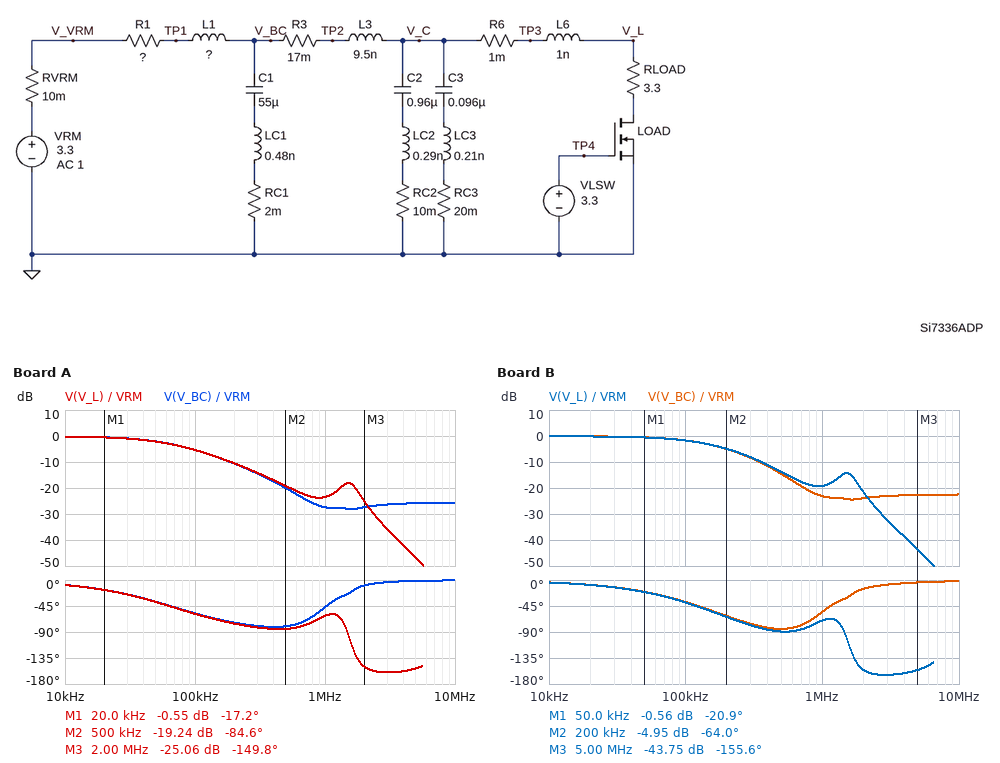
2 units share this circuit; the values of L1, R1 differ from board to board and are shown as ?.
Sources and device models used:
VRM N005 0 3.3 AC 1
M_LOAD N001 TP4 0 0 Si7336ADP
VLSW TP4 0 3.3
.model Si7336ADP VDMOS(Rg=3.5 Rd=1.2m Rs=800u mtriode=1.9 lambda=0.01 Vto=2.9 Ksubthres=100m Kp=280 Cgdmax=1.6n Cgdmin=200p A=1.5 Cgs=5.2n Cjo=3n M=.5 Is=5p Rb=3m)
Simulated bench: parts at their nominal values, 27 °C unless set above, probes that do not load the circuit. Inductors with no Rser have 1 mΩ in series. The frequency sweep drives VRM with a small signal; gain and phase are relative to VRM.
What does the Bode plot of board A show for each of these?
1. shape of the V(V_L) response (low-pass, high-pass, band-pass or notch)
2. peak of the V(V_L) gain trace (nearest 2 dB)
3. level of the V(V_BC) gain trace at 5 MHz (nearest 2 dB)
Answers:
low-pass
0 dB
-26 dB
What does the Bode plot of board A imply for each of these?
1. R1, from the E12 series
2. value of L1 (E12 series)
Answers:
0.033 Ω
8.2 nH
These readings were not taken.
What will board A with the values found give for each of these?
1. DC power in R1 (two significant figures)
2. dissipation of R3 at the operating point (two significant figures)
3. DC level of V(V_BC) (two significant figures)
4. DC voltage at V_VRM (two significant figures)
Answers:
32 mW
16 mW
3.3 V
3.3 V
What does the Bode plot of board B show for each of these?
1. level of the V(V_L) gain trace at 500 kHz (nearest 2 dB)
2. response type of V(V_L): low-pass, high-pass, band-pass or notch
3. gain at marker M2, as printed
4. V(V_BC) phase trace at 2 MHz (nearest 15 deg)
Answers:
-14 dB
low-pass
-4.95 dB
-15 deg
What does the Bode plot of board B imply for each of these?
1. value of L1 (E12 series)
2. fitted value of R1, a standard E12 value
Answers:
5.6 nH
0.01 Ω
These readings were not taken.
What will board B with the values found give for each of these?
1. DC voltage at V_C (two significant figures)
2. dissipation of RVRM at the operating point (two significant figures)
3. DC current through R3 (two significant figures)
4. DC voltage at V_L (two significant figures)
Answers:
3.3 V
9.7 mW
990 mA
3.3 V
